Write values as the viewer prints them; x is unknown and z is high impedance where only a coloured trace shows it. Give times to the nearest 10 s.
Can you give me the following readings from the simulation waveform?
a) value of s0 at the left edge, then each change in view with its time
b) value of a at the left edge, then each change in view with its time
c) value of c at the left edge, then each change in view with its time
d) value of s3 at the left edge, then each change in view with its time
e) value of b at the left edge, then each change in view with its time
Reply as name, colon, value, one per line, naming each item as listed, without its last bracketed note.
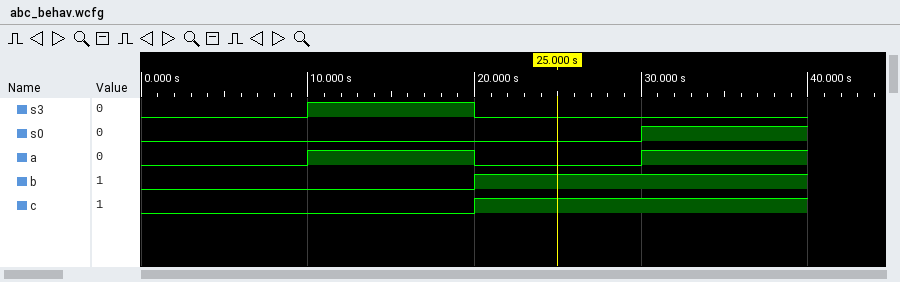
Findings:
value of s0 at the left edge, then each change in view with its time: 0, 1 at 30 s
value of a at the left edge, then each change in view with its time: 0, 1 at 10 s, 0 at 20 s, 1 at 30 s
value of c at the left edge, then each change in view with its time: 0, 1 at 20 s
value of s3 at the left edge, then each change in view with its time: 0, 1 at 10 s, 0 at 20 s
value of b at the left edge, then each change in view with its time: 0, 1 at 20 s
